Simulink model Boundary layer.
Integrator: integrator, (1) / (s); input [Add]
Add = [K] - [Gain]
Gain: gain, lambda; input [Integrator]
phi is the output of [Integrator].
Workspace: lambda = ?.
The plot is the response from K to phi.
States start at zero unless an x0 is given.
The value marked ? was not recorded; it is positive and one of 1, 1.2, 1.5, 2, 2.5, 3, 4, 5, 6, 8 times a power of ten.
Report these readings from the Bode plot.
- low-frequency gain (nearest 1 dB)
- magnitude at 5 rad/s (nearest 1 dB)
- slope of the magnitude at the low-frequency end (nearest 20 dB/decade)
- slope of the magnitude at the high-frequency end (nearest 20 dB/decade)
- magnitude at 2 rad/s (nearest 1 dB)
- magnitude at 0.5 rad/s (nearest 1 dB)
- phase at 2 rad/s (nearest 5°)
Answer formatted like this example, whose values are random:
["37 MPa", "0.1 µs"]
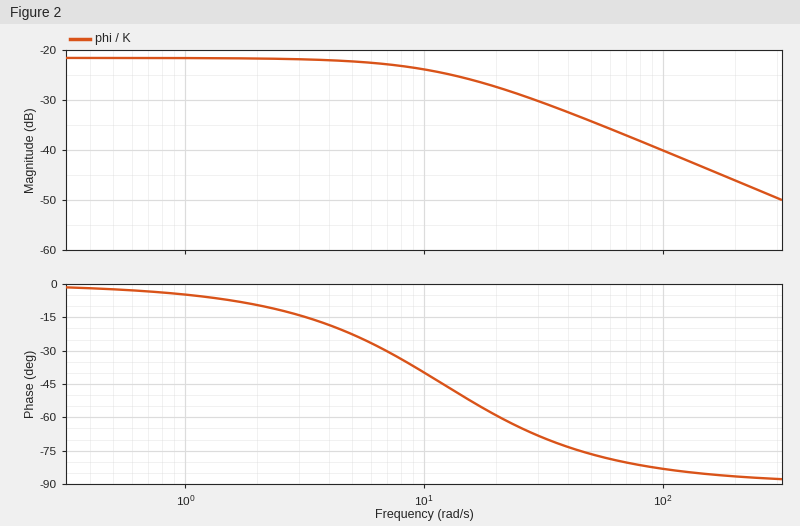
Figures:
["-22 dB", "-22 dB", "0 dB/decade", "-20 dB/decade", "-22 dB", "-22 dB", "-10°"]
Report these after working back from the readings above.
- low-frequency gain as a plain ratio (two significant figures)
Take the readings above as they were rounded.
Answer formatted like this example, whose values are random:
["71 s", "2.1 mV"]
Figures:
["0.079"]
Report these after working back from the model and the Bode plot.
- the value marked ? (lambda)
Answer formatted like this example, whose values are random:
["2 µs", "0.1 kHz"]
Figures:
["12"]
